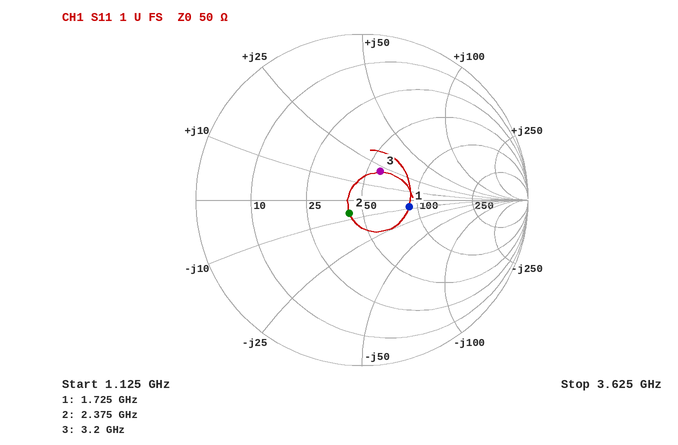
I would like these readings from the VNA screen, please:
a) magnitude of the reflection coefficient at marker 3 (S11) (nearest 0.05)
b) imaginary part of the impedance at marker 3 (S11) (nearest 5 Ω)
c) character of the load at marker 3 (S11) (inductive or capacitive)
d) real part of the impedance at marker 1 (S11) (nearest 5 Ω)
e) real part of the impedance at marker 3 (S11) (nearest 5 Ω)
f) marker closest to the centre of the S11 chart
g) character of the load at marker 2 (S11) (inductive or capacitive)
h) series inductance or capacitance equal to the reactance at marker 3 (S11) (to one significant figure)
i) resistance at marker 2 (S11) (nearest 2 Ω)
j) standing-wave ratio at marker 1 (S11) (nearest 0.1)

0.20
+20 Ω
inductive
90 Ω
60 Ω
marker 2
capacitive
1 nH
42 Ω
1.8
